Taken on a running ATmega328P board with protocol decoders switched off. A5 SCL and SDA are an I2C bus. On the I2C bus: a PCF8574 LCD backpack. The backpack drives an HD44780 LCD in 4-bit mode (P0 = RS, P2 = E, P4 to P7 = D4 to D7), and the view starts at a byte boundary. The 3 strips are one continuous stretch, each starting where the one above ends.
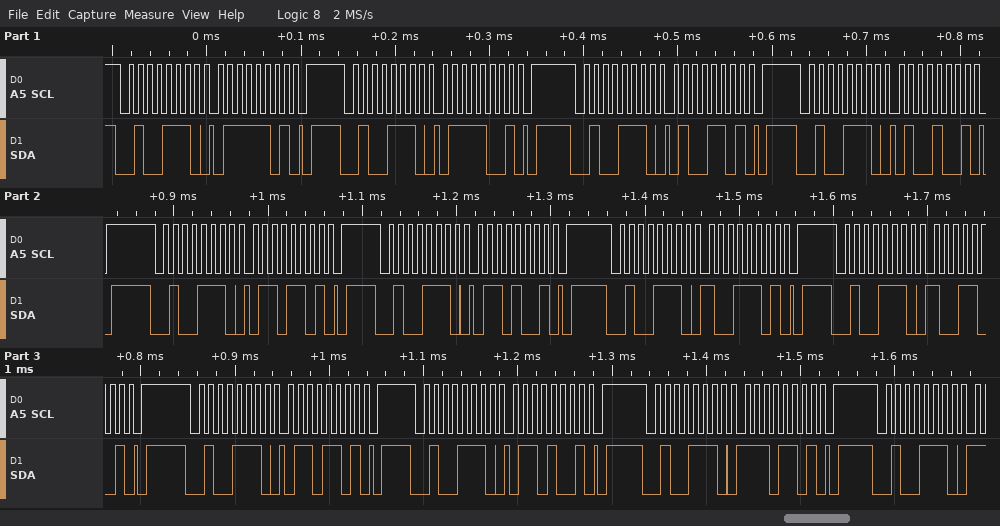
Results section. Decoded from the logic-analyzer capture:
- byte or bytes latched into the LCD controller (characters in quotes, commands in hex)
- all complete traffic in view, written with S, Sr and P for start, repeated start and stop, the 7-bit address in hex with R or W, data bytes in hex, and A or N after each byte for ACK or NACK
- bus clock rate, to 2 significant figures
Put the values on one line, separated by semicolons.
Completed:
't' 'i'; S 27W A 7D A P S 27W A 79 A P S 27W A 4D A P S 27W A 49 A P S 27W A 6D A P S 27W A 69 A P S 27W A 9D A P S 27W A 99 A P S 27W A 6D A P S 27W A 69 A P S 27W A ED A P S 27W A; 100 kHz
